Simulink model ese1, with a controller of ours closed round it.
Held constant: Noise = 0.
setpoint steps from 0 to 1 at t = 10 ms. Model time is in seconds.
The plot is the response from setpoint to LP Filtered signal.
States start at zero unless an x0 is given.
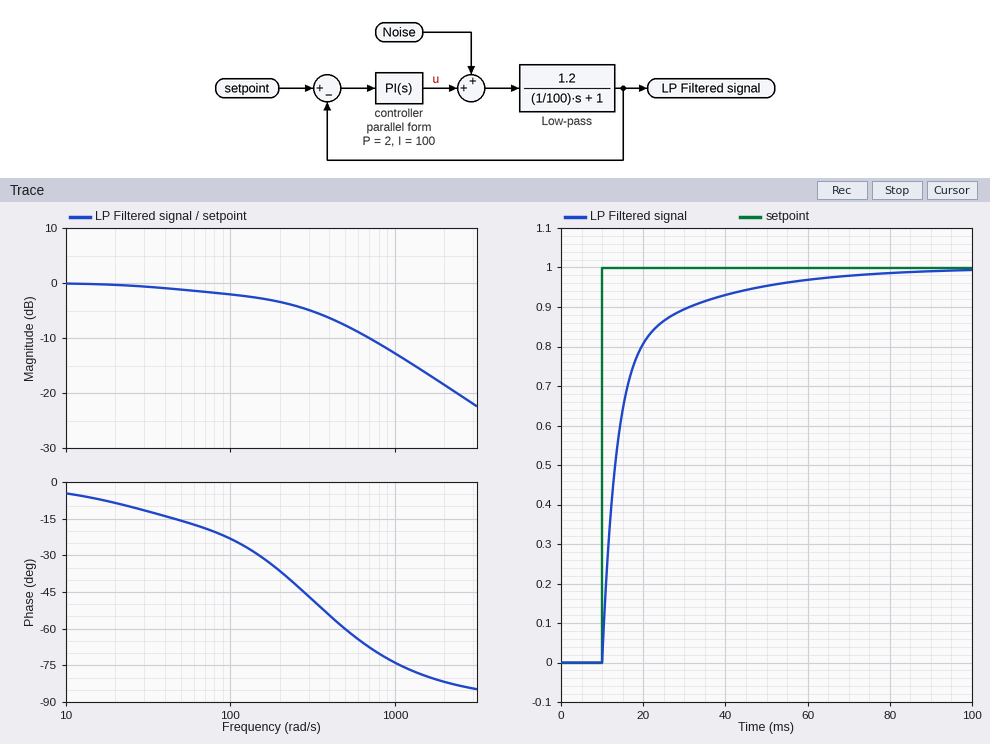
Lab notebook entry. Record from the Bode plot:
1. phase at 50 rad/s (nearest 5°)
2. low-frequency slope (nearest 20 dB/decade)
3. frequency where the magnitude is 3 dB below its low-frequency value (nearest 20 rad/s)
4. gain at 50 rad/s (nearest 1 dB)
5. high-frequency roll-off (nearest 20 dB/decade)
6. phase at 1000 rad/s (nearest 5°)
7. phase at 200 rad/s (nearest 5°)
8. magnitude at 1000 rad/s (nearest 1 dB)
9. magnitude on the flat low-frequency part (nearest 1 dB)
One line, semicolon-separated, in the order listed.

-15°; 0 dB/decade; 180 rad/s; -1 dB; -20 dB/decade; -75°; -35°; -13 dB; 0 dB
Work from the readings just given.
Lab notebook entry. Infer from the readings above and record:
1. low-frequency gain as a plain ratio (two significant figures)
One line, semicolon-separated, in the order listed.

1.0
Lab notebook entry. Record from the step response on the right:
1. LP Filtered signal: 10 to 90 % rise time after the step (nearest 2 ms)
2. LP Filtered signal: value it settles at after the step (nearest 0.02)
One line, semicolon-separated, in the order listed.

20 ms; 1.00
